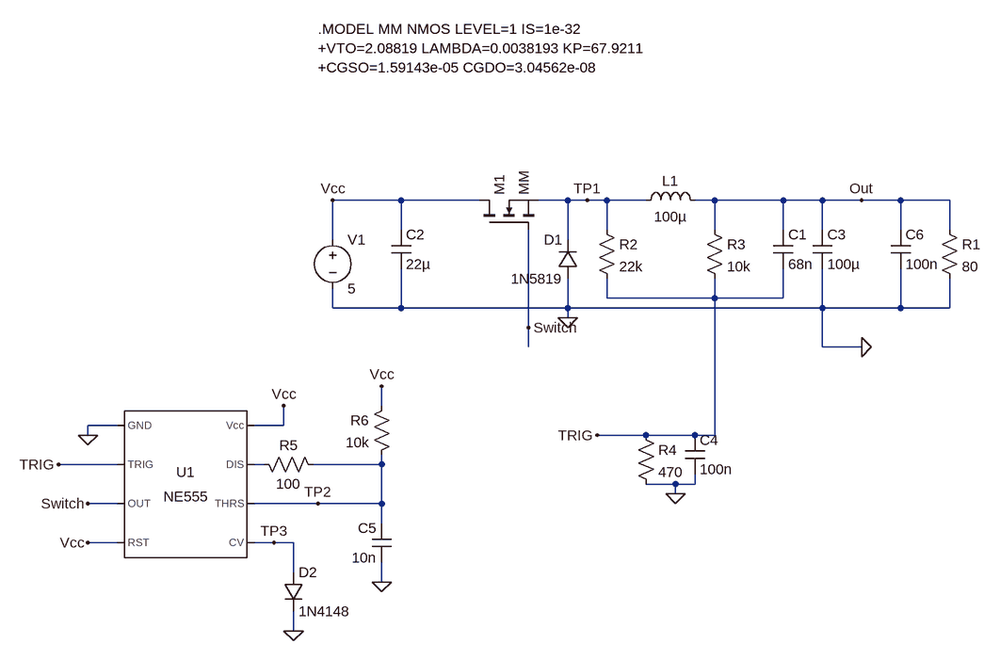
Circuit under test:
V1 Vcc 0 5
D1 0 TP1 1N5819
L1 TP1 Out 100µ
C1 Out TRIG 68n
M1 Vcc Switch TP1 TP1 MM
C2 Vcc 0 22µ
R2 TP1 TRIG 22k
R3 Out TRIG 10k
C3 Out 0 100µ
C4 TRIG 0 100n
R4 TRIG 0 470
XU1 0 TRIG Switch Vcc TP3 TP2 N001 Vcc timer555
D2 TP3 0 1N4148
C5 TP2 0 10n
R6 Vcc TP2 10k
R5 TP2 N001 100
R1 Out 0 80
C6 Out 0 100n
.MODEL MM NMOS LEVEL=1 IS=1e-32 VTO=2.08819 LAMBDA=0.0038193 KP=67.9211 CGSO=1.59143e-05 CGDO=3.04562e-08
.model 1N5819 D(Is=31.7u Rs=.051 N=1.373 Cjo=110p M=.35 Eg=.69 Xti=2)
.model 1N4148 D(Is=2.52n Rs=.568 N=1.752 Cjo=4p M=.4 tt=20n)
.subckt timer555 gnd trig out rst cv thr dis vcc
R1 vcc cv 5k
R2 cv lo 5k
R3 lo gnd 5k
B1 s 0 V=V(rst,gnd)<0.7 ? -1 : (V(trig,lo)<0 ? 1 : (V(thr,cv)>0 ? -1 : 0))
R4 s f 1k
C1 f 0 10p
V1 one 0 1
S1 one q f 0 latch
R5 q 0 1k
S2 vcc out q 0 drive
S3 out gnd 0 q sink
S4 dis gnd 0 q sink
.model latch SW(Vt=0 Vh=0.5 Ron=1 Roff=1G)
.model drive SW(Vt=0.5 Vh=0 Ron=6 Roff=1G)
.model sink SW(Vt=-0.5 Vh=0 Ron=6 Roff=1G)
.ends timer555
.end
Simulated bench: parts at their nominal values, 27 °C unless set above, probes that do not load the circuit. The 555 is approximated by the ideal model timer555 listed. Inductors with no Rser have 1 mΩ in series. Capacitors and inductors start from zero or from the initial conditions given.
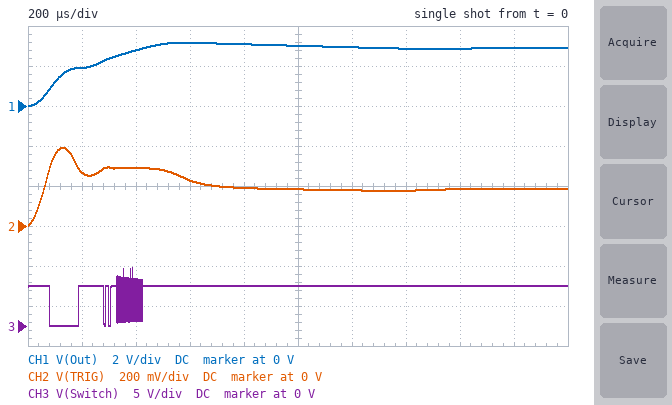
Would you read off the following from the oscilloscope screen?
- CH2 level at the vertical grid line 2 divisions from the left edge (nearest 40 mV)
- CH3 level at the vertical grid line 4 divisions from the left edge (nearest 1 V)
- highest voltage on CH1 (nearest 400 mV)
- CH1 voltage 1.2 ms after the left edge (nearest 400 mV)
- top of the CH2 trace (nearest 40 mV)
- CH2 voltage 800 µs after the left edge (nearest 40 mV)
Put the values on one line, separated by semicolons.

280 mV; 5 V; 3.2 V; 2.8 V; 400 mV; 200 mV
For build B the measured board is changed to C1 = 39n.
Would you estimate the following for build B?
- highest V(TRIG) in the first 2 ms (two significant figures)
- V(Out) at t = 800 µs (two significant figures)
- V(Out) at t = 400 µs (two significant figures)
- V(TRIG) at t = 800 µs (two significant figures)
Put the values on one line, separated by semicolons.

330 mV; 3.2 V; 3.3 V; 200 mV
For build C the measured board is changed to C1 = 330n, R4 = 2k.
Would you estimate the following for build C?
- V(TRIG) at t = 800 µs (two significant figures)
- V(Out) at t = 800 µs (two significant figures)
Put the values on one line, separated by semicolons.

420 mV; 1.1 V
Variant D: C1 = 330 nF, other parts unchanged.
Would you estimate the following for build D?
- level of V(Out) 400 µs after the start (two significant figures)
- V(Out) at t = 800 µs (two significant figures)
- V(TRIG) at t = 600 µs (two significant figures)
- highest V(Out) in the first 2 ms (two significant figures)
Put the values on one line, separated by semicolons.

1.3 V; 1.8 V; 290 mV; 2.9 V
